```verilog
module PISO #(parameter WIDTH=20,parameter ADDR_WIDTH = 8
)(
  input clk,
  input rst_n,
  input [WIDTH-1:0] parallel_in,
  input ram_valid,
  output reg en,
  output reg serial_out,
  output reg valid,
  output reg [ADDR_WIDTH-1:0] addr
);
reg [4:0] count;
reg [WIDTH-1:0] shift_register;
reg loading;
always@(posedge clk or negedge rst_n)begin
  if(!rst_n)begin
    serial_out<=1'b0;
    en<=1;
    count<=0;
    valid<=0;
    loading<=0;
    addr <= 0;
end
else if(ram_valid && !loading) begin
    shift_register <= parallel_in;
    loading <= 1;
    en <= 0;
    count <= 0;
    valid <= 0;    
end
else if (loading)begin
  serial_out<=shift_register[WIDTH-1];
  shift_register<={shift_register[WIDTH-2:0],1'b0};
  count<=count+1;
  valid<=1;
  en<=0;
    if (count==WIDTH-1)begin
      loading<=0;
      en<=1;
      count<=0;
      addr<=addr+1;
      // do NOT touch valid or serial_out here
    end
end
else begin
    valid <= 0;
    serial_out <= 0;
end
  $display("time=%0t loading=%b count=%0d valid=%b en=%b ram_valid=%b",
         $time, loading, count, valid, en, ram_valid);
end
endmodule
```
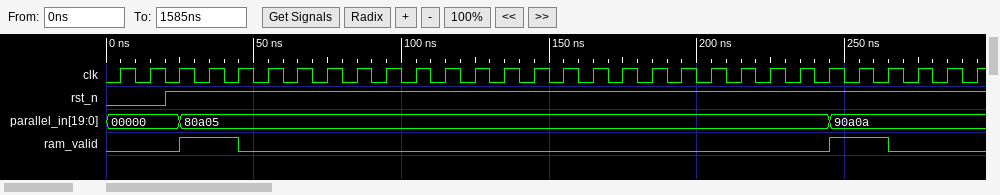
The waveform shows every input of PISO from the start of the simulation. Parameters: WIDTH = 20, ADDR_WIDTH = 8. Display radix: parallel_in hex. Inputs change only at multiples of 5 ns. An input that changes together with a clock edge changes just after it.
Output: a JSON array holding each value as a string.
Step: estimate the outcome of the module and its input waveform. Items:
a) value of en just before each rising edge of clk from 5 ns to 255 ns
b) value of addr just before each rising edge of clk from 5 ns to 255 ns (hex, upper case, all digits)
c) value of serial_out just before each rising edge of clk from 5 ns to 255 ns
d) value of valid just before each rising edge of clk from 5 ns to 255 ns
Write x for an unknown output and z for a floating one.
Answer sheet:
["1 1 1 1 0 0 0 0 0 0 0 0 0 0 0 0 0 0 0 0 0 0 0 0 1 1", "00, 00, 00, 00, 00, 00, 00, 00, 00, 00, 00, 00, 00, 00, 00, 00, 00, 00, 00, 00, 00, 00, 00, 00, 01, 01", "0 0 0 0 0 1 0 0 0 0 0 0 0 1 0 1 0 0 0 0 0 0 1 0 1 0", "0 0 0 0 0 1 1 1 1 1 1 1 1 1 1 1 1 1 1 1 1 1 1 1 1 0"]
